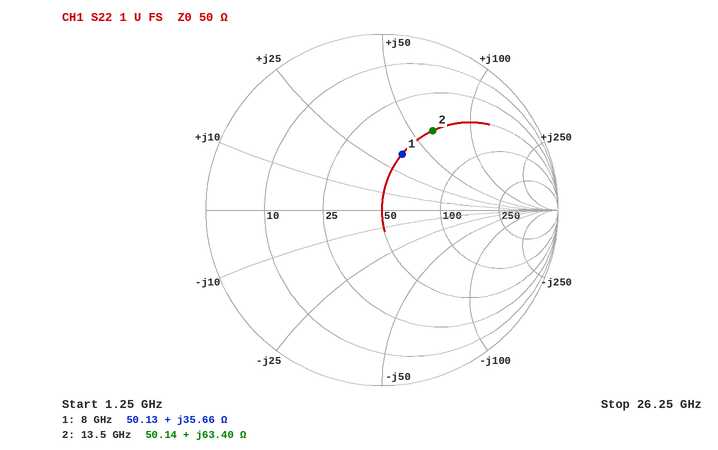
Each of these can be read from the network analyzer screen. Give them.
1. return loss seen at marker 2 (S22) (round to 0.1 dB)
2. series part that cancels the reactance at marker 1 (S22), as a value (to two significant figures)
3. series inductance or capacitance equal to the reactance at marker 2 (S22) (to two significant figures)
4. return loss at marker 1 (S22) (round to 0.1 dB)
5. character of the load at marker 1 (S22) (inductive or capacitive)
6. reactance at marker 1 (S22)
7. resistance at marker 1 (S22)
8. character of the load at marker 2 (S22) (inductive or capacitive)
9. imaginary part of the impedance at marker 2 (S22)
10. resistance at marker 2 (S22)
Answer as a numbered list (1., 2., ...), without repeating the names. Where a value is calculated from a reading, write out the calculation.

1. 5.4 dB
2. C = 1/(2π × 8 GHz × 35.66 Ω) ≈ 558 fF, so 560 fF to two significant figures
3. L = 63.4 Ω/(2π × 13.5 GHz) ≈ 747 pH, so 750 pH to two significant figures
4. 9.5 dB
5. inductive
6. +35.66 Ω
7. 50.13 Ω
8. inductive
9. +63.40 Ω
10. 50.14 Ω
